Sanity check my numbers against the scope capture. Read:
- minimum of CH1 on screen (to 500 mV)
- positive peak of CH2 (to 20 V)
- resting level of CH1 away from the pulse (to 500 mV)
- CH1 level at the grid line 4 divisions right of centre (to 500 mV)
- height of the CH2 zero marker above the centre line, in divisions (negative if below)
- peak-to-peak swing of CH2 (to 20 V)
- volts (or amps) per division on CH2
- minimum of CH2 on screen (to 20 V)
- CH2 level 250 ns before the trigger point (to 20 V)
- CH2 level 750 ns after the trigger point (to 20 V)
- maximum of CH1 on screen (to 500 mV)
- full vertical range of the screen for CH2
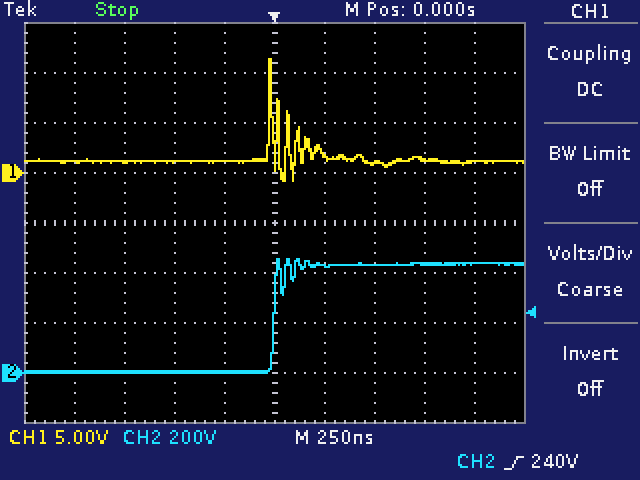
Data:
-1.0 V
460 V
1.0 V
1.0 V
-3.0 div
460 V
200 V
0 V
0 V
440 V
11.5 V
1.6 kV
